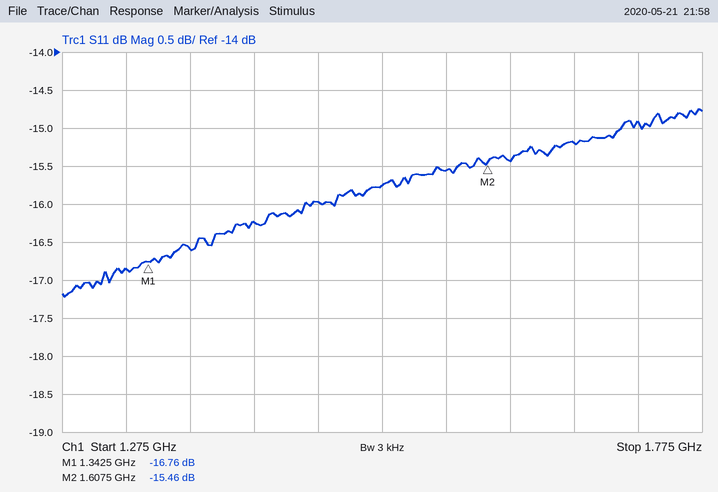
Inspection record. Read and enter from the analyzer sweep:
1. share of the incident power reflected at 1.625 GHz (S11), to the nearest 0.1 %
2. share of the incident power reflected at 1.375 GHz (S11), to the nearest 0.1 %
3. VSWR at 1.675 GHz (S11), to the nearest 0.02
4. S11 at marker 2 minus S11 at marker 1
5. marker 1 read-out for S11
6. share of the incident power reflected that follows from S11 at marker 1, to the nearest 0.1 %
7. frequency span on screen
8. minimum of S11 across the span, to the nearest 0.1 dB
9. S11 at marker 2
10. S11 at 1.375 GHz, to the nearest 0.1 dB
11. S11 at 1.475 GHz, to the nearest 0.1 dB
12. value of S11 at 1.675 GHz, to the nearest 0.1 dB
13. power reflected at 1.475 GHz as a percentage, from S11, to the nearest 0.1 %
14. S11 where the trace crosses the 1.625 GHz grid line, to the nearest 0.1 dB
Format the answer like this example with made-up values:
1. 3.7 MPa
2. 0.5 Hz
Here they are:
1. 2.9 %
2. 2.2 %
3. 1.42
4. 1.30 dB
5. -16.76 dB
6. 2.1 %
7. 500 MHz
8. -17.2 dB
9. -15.46 dB
10. -16.6 dB
11. -16.0 dB
12. -15.2 dB
13. 2.5 %
14. -15.4 dB
